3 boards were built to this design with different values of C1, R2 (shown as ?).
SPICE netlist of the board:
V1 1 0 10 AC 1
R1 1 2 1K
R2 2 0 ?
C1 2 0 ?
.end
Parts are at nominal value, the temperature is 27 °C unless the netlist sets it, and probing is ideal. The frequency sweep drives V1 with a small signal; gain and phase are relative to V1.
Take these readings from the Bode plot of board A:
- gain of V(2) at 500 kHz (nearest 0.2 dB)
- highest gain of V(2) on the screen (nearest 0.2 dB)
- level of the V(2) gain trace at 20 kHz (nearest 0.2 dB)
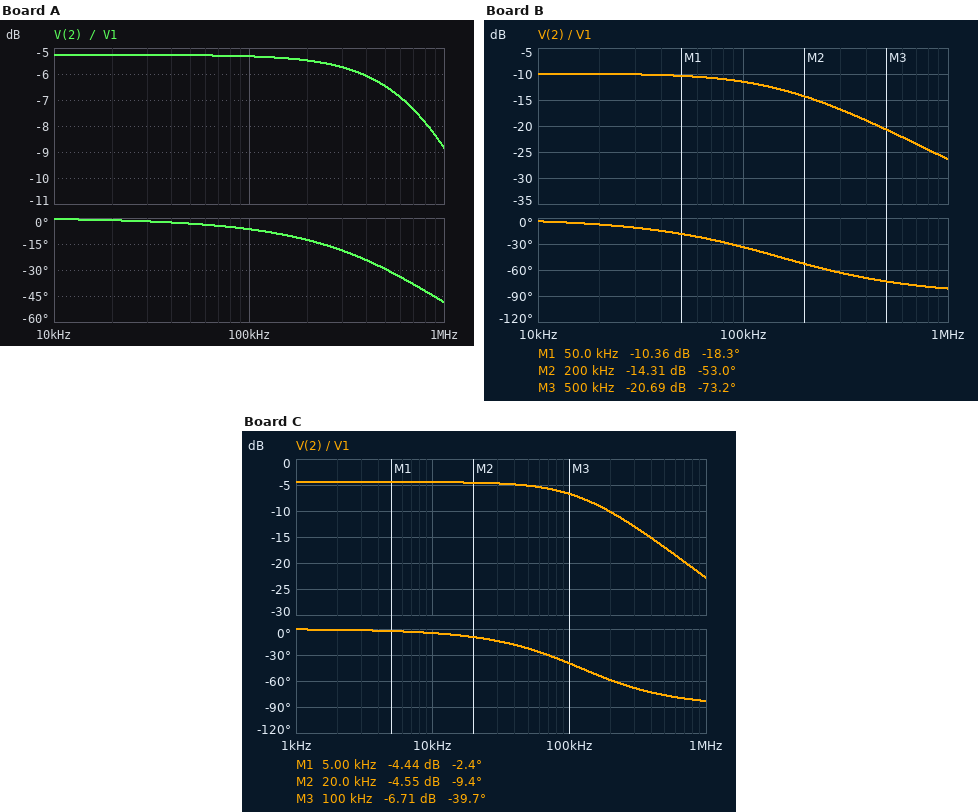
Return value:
-6.4 dB
-5.2 dB
-5.2 dB
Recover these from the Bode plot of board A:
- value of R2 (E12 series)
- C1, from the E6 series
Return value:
1.2 kΩ
330 pF
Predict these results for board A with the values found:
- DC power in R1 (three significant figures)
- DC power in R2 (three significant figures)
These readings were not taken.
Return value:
20.7 mW
24.8 mW
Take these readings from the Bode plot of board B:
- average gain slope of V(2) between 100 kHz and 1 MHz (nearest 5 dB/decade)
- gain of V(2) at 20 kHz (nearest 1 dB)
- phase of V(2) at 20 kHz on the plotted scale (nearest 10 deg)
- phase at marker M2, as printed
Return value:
-15 dB/decade
-10 dB
-10 deg
-53.0 deg
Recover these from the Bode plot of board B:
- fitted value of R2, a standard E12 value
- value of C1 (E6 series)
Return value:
470 Ω
3.3 nF
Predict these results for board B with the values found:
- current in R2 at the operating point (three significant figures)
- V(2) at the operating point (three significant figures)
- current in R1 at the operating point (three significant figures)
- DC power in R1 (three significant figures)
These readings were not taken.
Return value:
6.80 mA
3.20 V
6.80 mA
46.3 mW
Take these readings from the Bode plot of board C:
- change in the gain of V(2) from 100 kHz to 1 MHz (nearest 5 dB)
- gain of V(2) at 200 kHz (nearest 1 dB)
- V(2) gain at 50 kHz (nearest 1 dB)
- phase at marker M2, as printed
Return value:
-15 dB
-10 dB
-5 dB
-9.4 deg
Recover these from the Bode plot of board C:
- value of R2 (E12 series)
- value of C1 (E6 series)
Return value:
1.5 kΩ
2.2 nF
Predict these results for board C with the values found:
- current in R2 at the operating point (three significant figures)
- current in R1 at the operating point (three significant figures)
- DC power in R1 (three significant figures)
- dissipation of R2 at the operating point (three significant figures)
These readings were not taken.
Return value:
4.00 mA
4.00 mA
16.0 mW
24.0 mW
